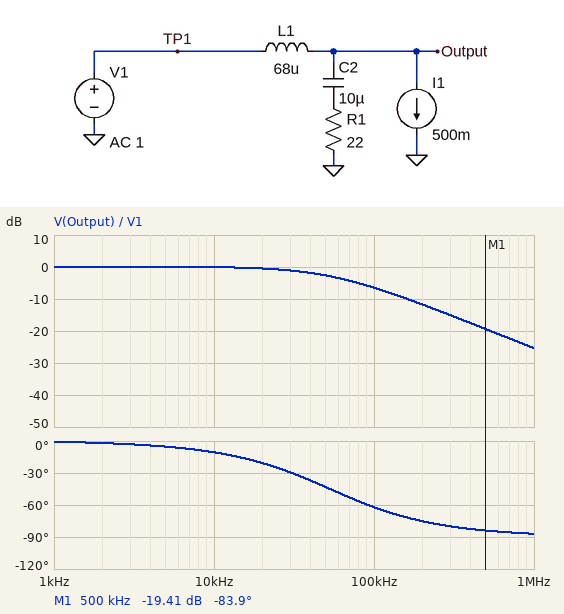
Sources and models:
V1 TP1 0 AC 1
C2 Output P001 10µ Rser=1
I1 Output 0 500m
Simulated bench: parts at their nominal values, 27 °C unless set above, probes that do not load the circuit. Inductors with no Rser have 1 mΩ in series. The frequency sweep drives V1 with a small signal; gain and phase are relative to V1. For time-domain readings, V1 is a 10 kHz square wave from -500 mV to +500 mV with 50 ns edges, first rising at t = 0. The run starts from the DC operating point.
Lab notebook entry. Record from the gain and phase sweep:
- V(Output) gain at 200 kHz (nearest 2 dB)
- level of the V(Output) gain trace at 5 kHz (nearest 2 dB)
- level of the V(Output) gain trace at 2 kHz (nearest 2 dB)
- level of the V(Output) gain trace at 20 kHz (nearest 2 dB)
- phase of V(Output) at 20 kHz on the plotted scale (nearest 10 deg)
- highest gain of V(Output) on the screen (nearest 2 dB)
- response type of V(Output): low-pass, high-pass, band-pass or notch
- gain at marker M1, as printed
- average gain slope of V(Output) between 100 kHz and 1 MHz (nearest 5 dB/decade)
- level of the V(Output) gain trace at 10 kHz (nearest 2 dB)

-12 dB
0 dB
0 dB
0 dB
-20 deg
0 dB
low-pass
-19.41 dB
-20 dB/decade
0 dB
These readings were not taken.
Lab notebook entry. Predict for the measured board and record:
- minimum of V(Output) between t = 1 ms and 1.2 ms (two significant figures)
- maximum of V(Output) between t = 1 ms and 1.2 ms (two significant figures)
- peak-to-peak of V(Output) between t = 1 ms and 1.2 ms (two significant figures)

-510 mV
510 mV
1.0 V
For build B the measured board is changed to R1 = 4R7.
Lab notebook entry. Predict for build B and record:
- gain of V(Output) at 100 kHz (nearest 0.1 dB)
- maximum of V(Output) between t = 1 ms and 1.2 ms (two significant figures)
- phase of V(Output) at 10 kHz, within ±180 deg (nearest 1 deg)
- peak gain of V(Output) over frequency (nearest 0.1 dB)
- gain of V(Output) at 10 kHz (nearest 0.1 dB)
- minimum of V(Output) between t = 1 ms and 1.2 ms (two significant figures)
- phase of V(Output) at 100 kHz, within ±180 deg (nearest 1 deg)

-17.5 dB
580 mV
-41 deg
1.1 dB
-0.5 dB
-580 mV
-84 deg
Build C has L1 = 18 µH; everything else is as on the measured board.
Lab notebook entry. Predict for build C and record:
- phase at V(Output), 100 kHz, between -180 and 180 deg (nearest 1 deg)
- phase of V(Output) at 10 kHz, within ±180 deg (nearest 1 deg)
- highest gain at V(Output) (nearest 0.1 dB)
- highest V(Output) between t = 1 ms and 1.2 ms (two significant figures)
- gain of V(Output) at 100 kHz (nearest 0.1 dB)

-26 deg
-3 deg
0 dB
500 mV
-0.9 dB
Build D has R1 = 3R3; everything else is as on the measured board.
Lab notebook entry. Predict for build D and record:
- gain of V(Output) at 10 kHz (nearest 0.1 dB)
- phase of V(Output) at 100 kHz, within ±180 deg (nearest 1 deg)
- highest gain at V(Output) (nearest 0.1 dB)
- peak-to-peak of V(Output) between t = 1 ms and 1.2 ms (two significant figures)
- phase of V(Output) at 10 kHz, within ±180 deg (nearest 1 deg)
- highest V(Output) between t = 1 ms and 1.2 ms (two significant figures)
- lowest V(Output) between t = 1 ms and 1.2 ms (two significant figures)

-0.9 dB
-86 deg
1.7 dB
1.2 V
-52 deg
600 mV
-600 mV
